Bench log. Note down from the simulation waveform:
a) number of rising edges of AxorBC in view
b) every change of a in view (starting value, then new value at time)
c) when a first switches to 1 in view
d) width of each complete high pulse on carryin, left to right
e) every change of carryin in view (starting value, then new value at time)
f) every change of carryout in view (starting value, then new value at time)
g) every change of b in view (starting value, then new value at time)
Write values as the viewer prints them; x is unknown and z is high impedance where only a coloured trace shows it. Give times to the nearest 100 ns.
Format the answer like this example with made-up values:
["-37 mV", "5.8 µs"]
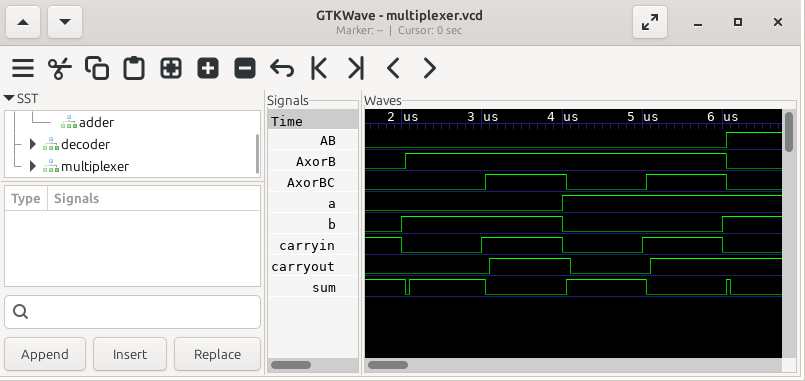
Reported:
["2", "0, 1 at 4000 ns", "4000 ns", "1000 ns, 1000 ns", "1, 0 at 2000 ns, 1 at 3000 ns, 0 at 4000 ns, 1 at 5000 ns, 0 at 6000 ns", "0, 1 at 3100 ns, 0 at 4100 ns, 1 at 5100 ns", "0, 1 at 2000 ns, 0 at 4000 ns, 1 at 6000 ns"]
